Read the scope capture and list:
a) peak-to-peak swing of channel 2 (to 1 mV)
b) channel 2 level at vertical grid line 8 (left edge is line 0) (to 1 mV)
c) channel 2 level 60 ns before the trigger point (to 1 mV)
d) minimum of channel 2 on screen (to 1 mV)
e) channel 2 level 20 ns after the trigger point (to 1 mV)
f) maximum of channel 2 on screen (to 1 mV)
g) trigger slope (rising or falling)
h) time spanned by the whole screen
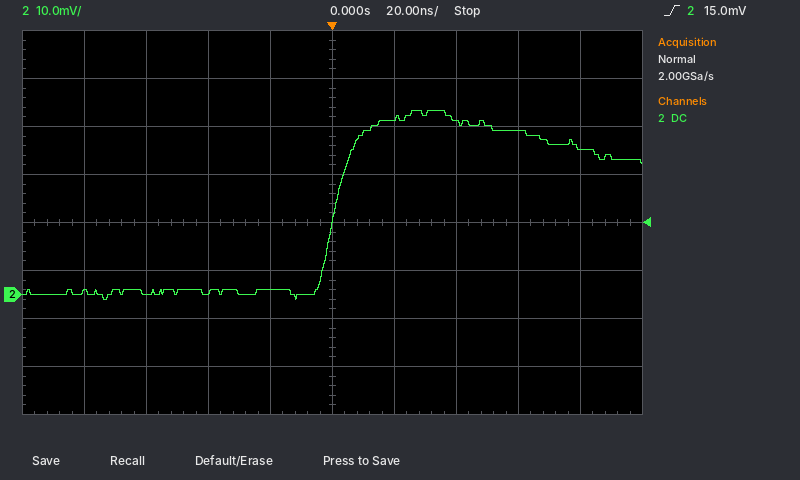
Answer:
39 mV
34 mV
0 mV
-1 mV
37 mV
38 mV
rising
200 ns
